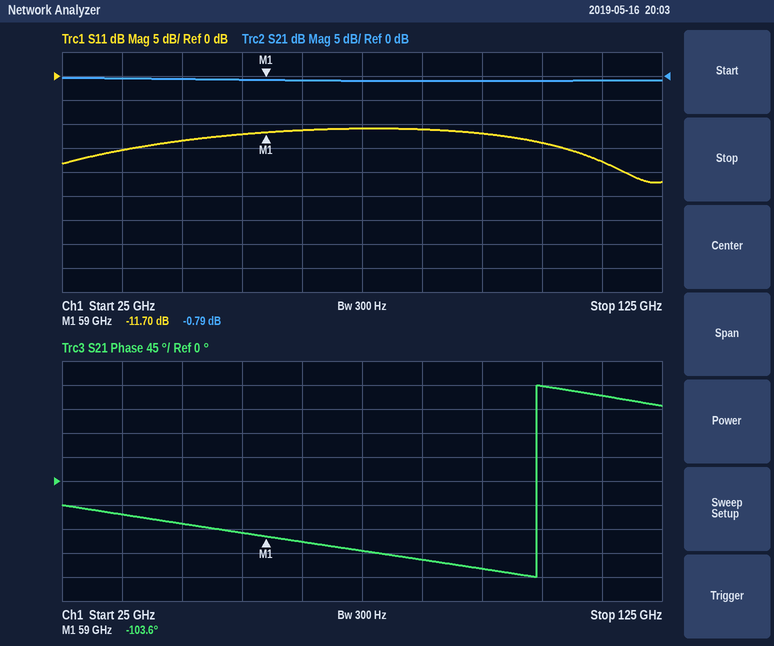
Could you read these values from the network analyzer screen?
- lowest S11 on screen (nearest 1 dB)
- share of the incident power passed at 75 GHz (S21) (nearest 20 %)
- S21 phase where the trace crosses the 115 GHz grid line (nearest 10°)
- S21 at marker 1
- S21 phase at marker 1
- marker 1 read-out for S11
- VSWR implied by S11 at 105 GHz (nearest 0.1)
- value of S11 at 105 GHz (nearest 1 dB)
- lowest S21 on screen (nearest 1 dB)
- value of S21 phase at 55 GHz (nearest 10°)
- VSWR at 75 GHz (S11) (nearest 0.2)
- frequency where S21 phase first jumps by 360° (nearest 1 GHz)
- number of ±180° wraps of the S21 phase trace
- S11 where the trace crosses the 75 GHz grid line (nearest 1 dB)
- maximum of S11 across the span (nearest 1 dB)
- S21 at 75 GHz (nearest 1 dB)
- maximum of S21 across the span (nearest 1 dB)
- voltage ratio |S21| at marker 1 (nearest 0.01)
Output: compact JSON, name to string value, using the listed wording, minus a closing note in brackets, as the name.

{"lowest S11 on screen": "-22 dB", "share of the incident power passed at 75 GHz (S21)": "80 %", "S21 phase where the trace crosses the 115 GHz grid line": "160°", "S21 at marker 1": "-0.79 dB", "S21 phase at marker 1": "-103.6°", "marker 1 read-out for S11": "-11.70 dB", "VSWR implied by S11 at 105 GHz": "1.5", "value of S11 at 105 GHz": "-14 dB", "lowest S21 on screen": "-1 dB", "value of S21 phase at 55 GHz": "-100°", "VSWR at 75 GHz (S11)": "1.8", "frequency where S21 phase first jumps by 360°": "104 GHz", "number of ±180° wraps of the S21 phase trace": "1", "S11 where the trace crosses the 75 GHz grid line": "-11 dB", "maximum of S11 across the span": "-11 dB", "S21 at 75 GHz": "-1 dB", "maximum of S21 across the span": "0 dB", "voltage ratio |S21| at marker 1": "0.91"}
